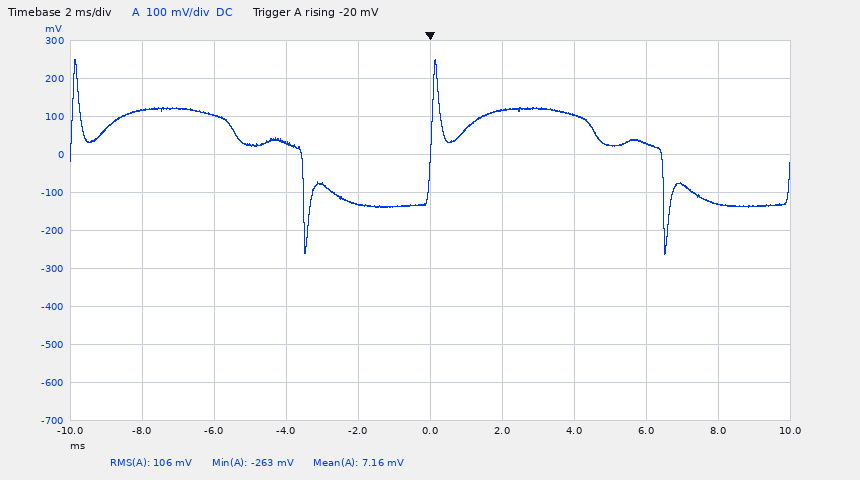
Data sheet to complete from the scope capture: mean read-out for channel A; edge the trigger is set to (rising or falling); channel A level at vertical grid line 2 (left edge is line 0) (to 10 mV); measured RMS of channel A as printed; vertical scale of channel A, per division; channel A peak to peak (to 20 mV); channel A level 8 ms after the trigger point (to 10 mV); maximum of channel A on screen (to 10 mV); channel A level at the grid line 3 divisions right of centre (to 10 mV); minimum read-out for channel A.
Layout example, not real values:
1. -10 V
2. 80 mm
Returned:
1. 7.16 mV
2. rising
3. 100 mV
4. 106 mV
5. 100 mV
6. 520 mV
7. -130 mV
8. 250 mV
9. 30 mV
10. -263 mV
